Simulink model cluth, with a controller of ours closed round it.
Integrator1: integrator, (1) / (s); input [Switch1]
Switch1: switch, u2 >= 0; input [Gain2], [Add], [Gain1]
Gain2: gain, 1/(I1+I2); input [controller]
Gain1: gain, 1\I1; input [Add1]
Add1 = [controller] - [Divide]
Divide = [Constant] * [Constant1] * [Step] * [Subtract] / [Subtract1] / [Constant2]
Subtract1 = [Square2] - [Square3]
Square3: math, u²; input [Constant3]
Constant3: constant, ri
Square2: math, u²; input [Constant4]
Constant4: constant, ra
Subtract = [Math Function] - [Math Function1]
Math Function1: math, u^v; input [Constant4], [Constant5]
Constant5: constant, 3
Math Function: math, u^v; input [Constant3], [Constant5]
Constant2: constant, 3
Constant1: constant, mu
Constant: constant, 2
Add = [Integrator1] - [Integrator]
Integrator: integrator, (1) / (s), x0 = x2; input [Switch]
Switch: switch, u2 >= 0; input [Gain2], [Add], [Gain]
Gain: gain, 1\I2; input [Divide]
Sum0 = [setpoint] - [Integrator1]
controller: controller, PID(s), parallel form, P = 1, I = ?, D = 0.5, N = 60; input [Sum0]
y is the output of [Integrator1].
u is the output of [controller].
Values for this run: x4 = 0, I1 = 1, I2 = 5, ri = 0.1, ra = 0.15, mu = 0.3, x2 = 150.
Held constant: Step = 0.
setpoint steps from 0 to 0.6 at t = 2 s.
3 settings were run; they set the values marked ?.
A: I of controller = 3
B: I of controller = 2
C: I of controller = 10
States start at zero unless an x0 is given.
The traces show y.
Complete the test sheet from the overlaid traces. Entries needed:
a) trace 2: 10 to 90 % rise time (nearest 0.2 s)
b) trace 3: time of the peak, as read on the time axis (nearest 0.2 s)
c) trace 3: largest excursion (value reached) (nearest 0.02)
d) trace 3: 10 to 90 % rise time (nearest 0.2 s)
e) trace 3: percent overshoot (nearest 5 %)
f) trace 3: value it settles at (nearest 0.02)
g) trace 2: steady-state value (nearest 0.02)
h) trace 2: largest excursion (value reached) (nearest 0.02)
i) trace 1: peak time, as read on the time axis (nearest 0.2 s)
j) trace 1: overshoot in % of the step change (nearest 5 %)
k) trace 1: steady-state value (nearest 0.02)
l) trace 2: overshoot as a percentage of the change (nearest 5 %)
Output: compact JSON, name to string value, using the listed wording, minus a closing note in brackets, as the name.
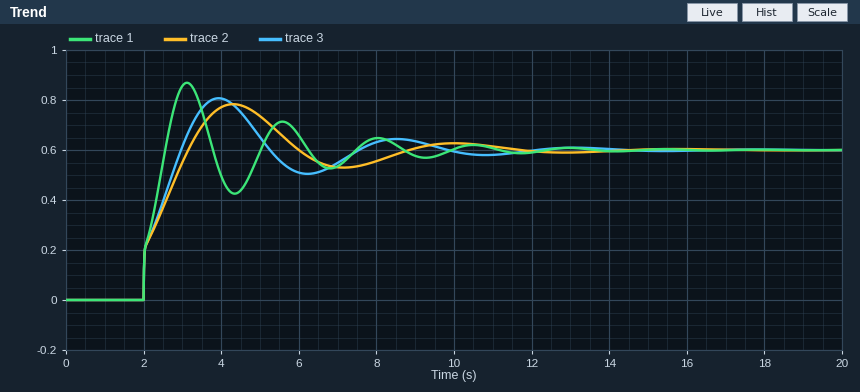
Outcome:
{"trace 2: 10 to 90 % rise time": "1.0 s", "trace 3: time of the peak, as read on the time axis": "4.0 s", "trace 3: largest excursion (value reached)": "0.80", "trace 3: 10 to 90 % rise time": "0.8 s", "trace 3: percent overshoot": "35 %", "trace 3: value it settles at": "0.60", "trace 2: steady-state value": "0.60", "trace 2: largest excursion (value reached)": "0.78", "trace 1: peak time, as read on the time axis": "3.2 s", "trace 1: overshoot in % of the step change": "45 %", "trace 1: steady-state value": "0.60", "trace 2: overshoot as a percentage of the change": "30 %"}
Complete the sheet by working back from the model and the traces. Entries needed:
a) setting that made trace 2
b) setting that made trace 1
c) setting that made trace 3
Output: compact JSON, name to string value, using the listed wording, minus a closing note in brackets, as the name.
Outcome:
{"setting that made trace 2": "B", "setting that made trace 1": "C", "setting that made trace 3": "A"}
